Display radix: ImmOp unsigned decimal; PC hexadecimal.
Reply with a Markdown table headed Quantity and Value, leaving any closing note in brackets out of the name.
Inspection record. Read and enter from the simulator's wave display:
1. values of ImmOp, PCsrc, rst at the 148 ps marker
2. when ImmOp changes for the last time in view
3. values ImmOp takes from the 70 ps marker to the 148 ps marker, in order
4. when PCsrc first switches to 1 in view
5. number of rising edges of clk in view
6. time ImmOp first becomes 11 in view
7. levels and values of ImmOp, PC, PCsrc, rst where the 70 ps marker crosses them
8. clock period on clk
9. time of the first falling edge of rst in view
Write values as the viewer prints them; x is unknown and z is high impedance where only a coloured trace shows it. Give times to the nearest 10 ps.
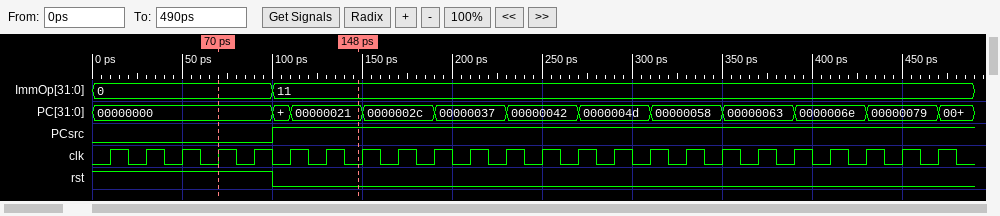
| Quantity | Value |
|---|---|
| values of ImmOp, PCsrc, rst at the 148 ps marker | ImmOp=11, PCsrc=1, rst=0 |
| when ImmOp changes for the last time in view | 100 ps |
| values ImmOp takes from the 70 ps marker to the 148 ps marker, in order | 0, 11 |
| when PCsrc first switches to 1 in view | 100 ps |
| number of rising edges of clk in view | 24 |
| time ImmOp first becomes 11 in view | 100 ps |
| levels and values of ImmOp, PC, PCsrc, rst where the 70 ps marker crosses them | ImmOp=0, PC=00000000, PCsrc=0, rst=1 |
| clock period on clk | 20 ps |
| time of the first falling edge of rst in view | 100 ps |
